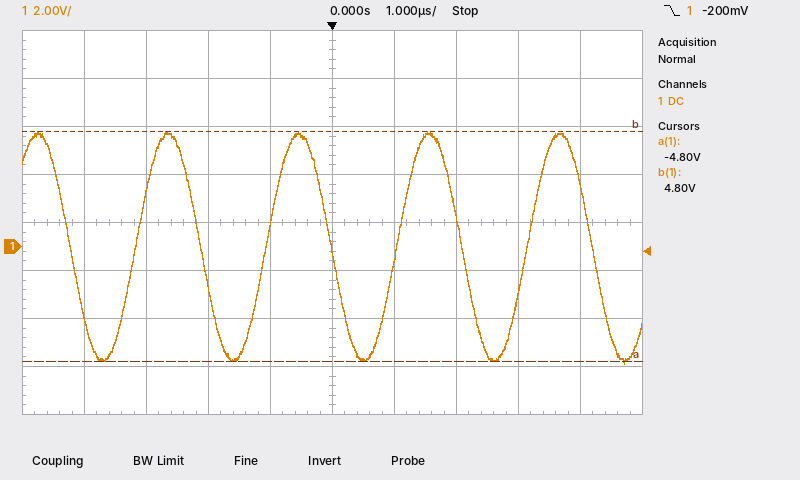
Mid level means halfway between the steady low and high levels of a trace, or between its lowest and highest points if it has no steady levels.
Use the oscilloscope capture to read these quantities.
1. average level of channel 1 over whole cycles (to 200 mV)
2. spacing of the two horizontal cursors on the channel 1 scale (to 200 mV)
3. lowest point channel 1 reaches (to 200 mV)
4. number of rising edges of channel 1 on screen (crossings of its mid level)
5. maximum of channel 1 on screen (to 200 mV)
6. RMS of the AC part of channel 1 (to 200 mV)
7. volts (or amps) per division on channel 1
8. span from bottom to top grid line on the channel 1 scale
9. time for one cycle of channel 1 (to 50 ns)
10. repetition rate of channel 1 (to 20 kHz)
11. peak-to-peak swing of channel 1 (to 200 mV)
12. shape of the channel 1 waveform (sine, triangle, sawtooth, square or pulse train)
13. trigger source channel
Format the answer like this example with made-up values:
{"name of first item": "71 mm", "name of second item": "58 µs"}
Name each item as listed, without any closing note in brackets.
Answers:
{"average level of channel 1 over whole cycles": "0.0 V", "spacing of the two horizontal cursors on the channel 1 scale": "9.6 V", "lowest point channel 1 reaches": "-4.8 V", "number of rising edges of channel 1 on screen": "4", "maximum of channel 1 on screen": "4.8 V", "RMS of the AC part of channel 1": "3.4 V", "volts (or amps) per division on channel 1": "2 V", "span from bottom to top grid line on the channel 1 scale": "16 V", "time for one cycle of channel 1": "2.10 µs", "repetition rate of channel 1": "480 kHz", "peak-to-peak swing of channel 1": "9.6 V", "shape of the channel 1 waveform": "sine", "trigger source channel": "channel 1"}
